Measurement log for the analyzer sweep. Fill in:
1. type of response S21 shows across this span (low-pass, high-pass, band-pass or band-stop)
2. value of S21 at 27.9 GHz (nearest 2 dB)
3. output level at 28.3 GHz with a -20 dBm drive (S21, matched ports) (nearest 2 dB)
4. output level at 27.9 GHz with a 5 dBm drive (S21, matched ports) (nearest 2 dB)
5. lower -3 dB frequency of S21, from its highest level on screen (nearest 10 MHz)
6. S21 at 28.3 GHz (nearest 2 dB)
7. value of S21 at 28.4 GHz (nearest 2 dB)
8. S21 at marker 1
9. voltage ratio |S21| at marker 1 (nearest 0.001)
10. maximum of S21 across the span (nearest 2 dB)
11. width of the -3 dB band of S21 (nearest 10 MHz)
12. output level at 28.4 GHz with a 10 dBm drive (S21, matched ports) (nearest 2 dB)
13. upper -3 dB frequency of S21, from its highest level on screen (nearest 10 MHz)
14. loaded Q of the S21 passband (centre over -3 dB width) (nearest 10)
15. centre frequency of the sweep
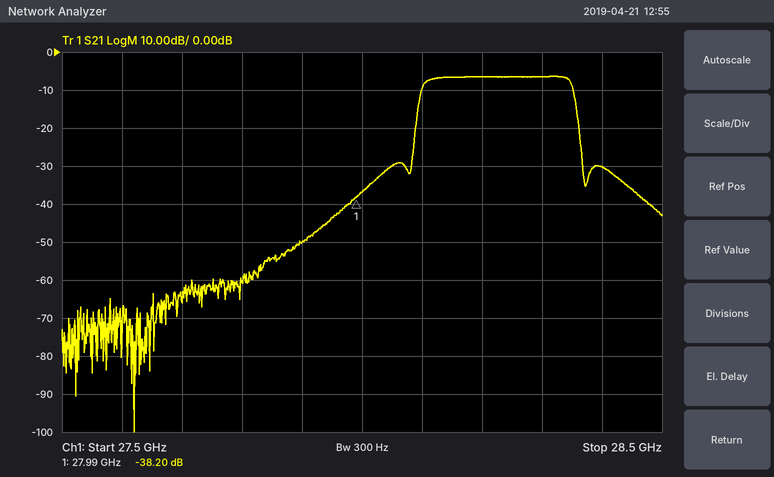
band-pass
-50 dB
-26 dBm
-44 dBm
28.10 GHz
-6 dB
-30 dB
-38.20 dB
0.012
-6 dB
250 MHz
-20 dBm
28.35 GHz
110
28 GHz
